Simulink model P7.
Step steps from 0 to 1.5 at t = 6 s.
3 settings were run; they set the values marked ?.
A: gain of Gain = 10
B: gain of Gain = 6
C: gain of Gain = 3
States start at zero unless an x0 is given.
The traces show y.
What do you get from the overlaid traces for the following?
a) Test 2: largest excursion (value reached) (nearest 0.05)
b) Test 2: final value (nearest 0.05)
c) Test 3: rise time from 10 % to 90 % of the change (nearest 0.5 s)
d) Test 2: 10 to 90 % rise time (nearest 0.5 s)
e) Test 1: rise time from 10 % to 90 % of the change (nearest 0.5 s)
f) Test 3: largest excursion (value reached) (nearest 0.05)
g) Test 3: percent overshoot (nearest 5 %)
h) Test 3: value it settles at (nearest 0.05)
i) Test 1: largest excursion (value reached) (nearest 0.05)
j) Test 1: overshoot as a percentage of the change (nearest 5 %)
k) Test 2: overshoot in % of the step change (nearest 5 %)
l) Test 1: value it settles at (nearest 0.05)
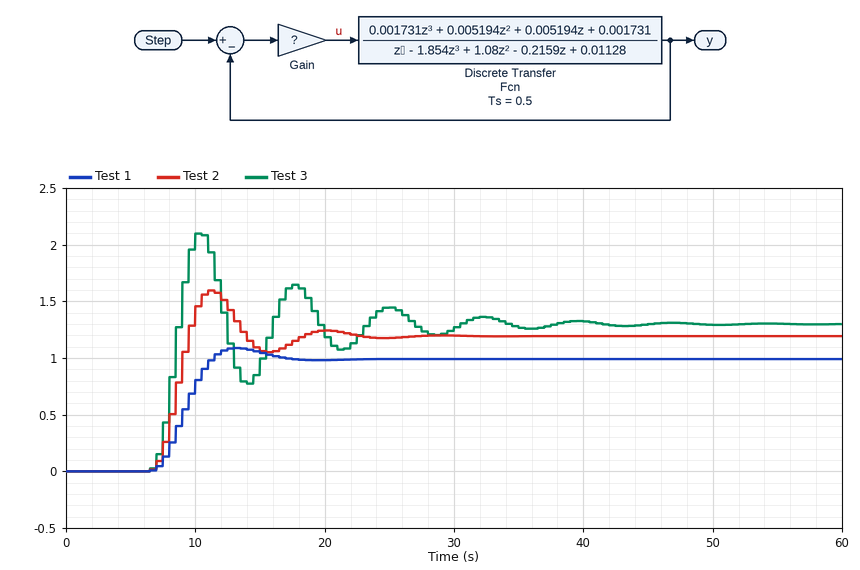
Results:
1.60
1.20
1.5 s
2.0 s
3.0 s
2.10
60 %
1.30
1.10
10 %
35 %
1.00
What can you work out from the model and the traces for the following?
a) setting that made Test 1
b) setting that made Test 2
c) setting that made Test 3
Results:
C
B
A
